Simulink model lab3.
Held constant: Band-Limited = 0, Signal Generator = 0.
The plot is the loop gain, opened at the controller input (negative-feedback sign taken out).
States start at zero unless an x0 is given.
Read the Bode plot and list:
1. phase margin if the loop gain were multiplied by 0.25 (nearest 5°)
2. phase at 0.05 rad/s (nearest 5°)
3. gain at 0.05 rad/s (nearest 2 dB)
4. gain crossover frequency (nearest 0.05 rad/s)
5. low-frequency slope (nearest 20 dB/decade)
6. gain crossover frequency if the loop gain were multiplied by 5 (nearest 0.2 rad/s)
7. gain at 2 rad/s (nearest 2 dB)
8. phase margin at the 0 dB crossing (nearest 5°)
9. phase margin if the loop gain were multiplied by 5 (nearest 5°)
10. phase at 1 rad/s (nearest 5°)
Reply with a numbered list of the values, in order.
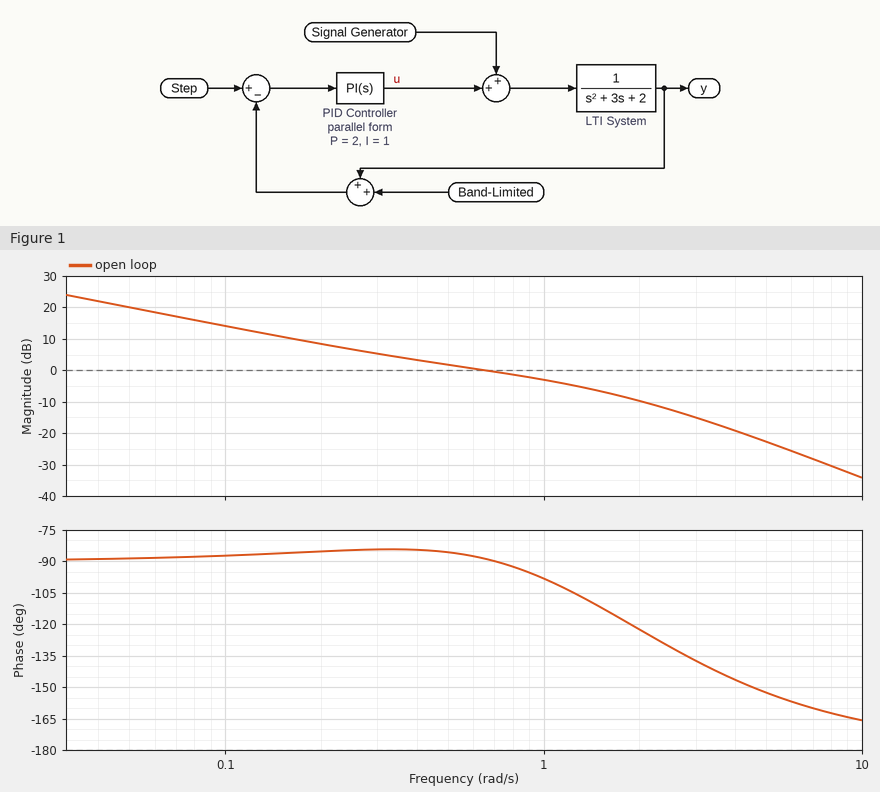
1. 95°
2. -90°
3. 20 dB
4. 0.65 rad/s
5. -20 dB/decade
6. 2.8 rad/s
7. -10 dB
8. 90°
9. 45°
10. -100°
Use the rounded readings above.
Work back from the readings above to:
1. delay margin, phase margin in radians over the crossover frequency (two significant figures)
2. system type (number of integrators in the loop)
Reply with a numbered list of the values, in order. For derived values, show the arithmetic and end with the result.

1. 90 × π / 180 / 0.65 = 2.4 s
2. 1
